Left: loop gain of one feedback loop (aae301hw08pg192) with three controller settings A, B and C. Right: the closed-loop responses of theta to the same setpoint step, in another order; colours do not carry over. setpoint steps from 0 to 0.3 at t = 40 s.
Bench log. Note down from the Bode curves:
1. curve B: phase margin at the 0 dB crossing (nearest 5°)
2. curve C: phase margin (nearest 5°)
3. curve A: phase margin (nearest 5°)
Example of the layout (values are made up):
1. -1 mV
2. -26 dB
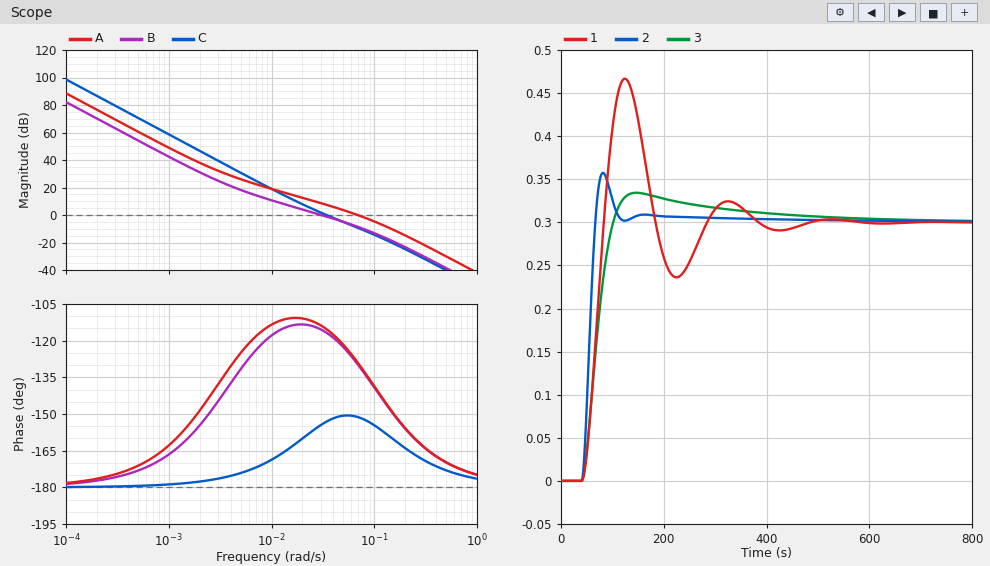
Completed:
1. 65°
2. 25°
3. 50°
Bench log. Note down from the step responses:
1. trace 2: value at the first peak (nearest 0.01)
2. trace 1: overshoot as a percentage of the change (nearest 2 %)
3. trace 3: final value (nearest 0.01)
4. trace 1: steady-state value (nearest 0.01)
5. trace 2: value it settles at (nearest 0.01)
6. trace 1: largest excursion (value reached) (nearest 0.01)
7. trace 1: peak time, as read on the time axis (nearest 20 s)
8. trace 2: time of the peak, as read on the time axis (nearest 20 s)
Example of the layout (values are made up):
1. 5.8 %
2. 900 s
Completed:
1. 0.36
2. 56 %
3. 0.30
4. 0.30
5. 0.30
6. 0.47
7. 120 s
8. 80 s
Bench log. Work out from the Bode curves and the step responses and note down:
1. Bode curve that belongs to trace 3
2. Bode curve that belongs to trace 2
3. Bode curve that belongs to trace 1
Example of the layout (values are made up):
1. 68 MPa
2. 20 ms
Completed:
1. B
2. A
3. C
